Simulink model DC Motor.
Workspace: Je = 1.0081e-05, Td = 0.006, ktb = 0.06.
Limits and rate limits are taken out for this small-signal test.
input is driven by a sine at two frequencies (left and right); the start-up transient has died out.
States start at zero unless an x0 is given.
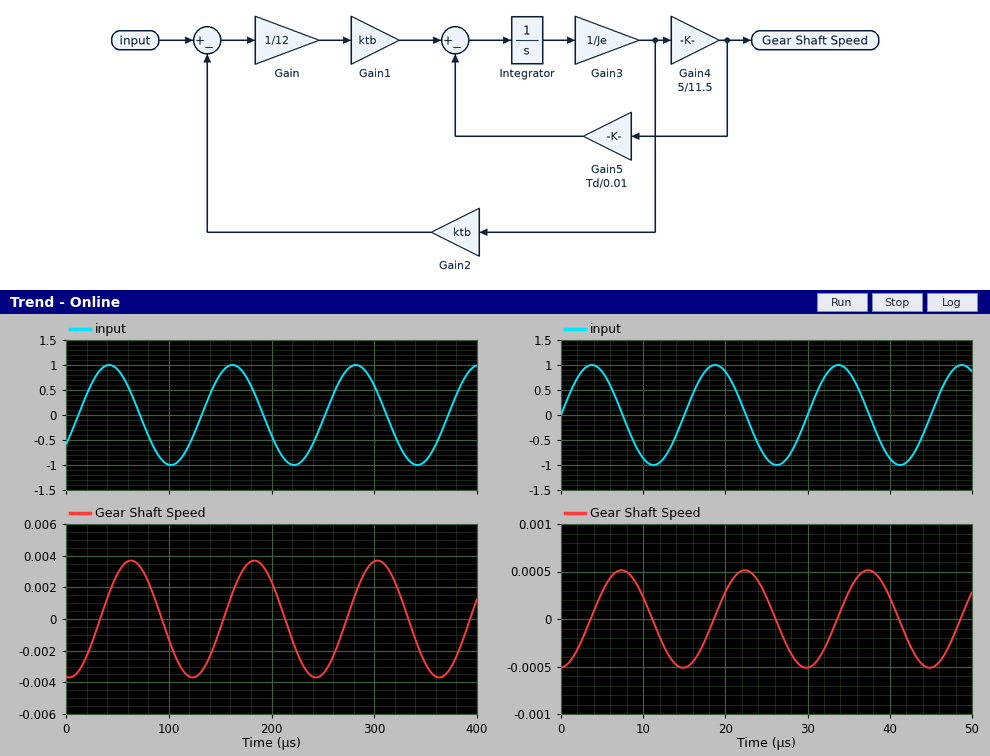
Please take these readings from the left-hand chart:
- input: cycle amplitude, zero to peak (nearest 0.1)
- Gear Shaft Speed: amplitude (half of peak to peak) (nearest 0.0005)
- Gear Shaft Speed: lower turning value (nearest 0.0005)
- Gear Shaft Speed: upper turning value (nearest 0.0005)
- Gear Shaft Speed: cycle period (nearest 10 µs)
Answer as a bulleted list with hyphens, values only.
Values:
- 1.0
- 0.0035
- -0.0035
- 0.0035
- 120 µs
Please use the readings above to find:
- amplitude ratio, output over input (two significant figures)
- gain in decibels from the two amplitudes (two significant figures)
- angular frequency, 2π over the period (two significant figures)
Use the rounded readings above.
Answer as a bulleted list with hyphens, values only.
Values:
- 0.0035
- -49 dB
- 0.052 rad/µs
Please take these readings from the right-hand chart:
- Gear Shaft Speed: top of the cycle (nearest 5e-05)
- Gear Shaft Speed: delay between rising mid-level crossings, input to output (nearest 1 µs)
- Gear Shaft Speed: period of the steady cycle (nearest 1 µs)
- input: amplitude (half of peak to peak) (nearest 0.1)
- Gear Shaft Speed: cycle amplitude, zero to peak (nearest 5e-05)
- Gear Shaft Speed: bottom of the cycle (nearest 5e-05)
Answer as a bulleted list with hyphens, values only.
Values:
- 0.00050
- 4 µs
- 15 µs
- 1.0
- 0.00050
- -0.00050
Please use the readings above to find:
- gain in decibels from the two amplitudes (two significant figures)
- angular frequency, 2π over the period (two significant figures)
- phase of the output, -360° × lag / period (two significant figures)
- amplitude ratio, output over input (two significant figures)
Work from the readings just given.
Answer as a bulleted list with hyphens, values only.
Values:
- -66 dB
- 0.42 rad/µs
- -96°
- 0.00050
